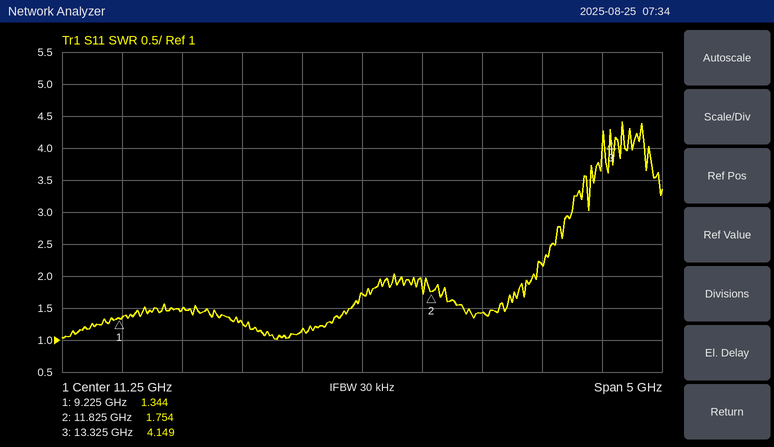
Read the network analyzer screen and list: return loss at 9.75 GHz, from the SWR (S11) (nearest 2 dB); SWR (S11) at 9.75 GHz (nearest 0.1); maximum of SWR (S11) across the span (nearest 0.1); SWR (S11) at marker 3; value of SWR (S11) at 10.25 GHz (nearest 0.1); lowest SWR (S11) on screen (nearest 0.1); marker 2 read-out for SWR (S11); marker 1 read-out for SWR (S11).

14 dB
1.5
4.4
4.149
1.3
1.0
1.754
1.344
